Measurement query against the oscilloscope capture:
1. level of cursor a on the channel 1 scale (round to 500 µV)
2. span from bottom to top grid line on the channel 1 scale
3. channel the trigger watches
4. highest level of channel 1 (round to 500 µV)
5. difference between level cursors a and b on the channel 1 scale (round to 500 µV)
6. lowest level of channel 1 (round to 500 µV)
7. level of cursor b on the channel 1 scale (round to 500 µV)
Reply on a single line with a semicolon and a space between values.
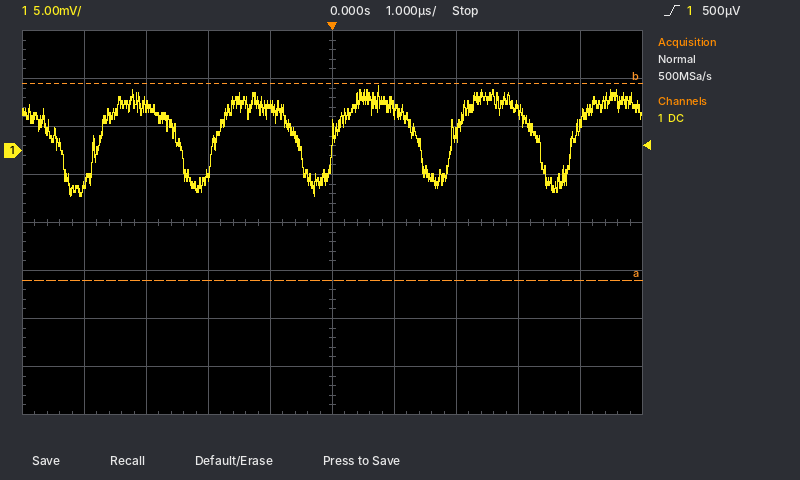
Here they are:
-13.5 mV; 40 mV; channel 1; 7.0 mV; 20.5 mV; -5.0 mV; 7.0 mV
